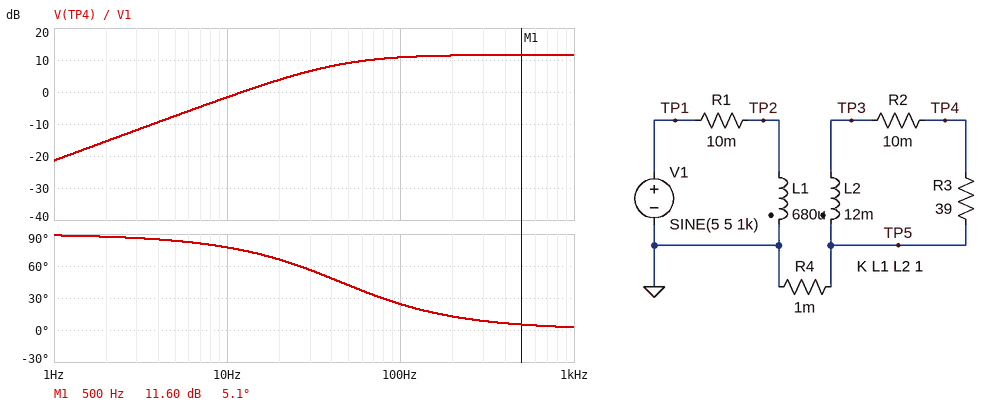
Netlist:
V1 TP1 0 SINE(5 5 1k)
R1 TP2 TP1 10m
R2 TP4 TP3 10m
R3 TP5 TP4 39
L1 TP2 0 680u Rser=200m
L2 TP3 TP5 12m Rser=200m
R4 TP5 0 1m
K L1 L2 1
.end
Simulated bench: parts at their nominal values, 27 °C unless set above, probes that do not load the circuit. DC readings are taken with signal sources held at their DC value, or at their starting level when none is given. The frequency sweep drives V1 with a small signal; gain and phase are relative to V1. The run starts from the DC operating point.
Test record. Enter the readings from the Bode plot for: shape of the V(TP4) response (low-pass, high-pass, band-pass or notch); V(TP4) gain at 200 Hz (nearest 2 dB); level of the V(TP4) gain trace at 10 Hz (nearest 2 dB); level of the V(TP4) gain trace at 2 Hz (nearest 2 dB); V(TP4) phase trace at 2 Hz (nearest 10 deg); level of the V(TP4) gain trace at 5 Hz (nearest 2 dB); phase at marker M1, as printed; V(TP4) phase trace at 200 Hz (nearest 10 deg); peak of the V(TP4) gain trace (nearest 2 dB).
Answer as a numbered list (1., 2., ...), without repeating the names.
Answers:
1. high-pass
2. 12 dB
3. -2 dB
4. -16 dB
5. 90 deg
6. -8 dB
7. 5.1 deg
8. 10 deg
9. 12 dB
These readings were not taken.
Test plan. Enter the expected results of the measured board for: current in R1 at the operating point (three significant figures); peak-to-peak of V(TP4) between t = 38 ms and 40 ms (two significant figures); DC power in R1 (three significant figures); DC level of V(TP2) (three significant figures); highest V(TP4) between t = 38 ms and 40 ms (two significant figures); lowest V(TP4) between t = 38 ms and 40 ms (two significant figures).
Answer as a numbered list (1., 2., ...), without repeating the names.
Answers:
1. 23.8 A
2. 38 V
3. 5.67 W
4. 4.76 V
5. 19 V
6. -19 V
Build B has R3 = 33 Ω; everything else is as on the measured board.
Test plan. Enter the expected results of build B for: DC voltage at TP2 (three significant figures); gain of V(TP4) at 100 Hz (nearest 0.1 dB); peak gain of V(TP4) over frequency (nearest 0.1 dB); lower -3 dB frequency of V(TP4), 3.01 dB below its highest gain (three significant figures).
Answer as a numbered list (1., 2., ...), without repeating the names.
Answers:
1. 4.76 V
2. 10.7 dB
3. 11.5 dB
4. 44.2 Hz
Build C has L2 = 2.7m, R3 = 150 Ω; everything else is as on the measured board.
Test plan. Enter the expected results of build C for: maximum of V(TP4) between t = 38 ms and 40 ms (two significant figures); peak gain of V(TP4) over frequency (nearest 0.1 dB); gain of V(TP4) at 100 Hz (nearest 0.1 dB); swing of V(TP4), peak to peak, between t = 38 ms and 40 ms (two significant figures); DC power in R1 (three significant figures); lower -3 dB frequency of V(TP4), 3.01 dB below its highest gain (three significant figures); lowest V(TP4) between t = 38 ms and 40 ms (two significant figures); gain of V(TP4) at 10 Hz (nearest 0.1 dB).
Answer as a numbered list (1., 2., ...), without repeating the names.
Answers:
1. 9.9 V
2. 5.9 dB
3. 5.0 dB
4. 20 V
5. 5.67 W
6. 48.9 Hz
7. -9.9 V
8. -8.0 dB
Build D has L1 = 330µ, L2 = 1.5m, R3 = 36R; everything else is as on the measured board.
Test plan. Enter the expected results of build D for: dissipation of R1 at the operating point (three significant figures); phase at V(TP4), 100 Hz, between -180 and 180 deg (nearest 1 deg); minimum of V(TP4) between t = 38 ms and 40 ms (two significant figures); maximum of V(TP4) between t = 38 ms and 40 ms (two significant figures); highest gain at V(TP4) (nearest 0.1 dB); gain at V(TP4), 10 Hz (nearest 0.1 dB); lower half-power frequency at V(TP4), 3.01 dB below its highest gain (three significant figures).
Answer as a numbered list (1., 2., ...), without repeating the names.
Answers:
1. 5.67 W
2. 45 deg
3. -10 V
4. 10 V
5. 6.3 dB
6. -13.6 dB
7. 98.7 Hz
